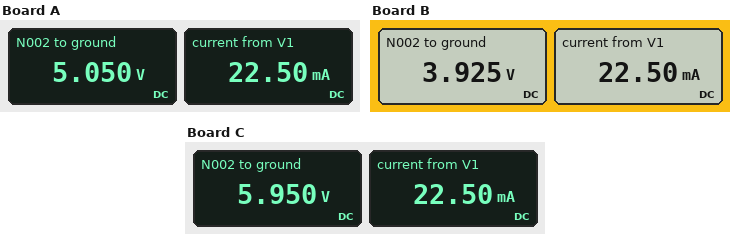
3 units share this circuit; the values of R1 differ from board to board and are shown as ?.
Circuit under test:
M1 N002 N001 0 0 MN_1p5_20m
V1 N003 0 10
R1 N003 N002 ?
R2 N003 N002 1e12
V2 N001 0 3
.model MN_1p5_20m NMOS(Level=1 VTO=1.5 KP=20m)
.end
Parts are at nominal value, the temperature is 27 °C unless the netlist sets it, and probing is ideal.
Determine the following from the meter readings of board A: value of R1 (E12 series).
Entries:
220 Ω
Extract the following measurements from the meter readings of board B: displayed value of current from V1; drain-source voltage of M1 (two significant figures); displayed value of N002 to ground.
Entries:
22.50 mA
3.9 V
3.925 V
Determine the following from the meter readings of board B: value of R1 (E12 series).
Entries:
270 Ω
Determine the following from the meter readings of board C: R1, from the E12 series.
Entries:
180 Ω
